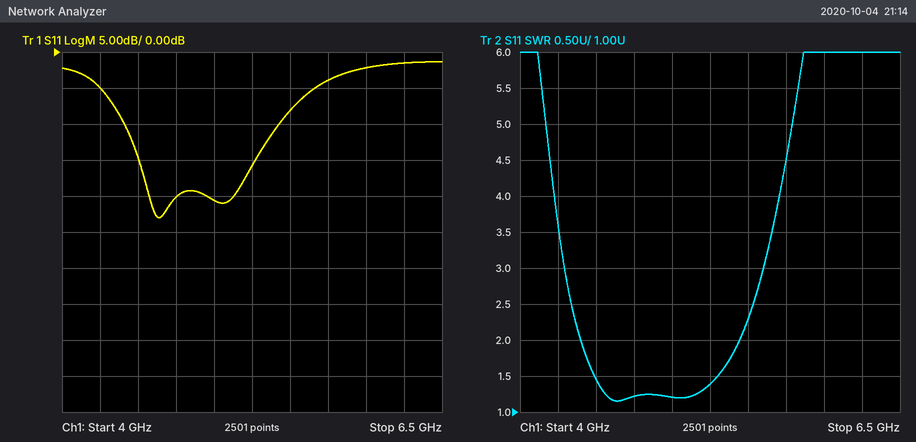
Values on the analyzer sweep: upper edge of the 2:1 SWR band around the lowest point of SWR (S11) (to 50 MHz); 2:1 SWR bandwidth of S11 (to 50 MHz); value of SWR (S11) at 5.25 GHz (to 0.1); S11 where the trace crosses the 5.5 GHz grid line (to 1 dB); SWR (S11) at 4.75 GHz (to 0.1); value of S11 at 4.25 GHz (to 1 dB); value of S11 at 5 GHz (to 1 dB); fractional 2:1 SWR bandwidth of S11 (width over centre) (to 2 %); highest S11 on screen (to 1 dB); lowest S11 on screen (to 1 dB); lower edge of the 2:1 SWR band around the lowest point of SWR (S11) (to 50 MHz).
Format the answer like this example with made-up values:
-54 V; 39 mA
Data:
5.45 GHz; 1.05 GHz; 1.4; -8 dB; 1.2; -5 dB; -21 dB; 22 %; -1 dB; -23 dB; 4.40 GHz
